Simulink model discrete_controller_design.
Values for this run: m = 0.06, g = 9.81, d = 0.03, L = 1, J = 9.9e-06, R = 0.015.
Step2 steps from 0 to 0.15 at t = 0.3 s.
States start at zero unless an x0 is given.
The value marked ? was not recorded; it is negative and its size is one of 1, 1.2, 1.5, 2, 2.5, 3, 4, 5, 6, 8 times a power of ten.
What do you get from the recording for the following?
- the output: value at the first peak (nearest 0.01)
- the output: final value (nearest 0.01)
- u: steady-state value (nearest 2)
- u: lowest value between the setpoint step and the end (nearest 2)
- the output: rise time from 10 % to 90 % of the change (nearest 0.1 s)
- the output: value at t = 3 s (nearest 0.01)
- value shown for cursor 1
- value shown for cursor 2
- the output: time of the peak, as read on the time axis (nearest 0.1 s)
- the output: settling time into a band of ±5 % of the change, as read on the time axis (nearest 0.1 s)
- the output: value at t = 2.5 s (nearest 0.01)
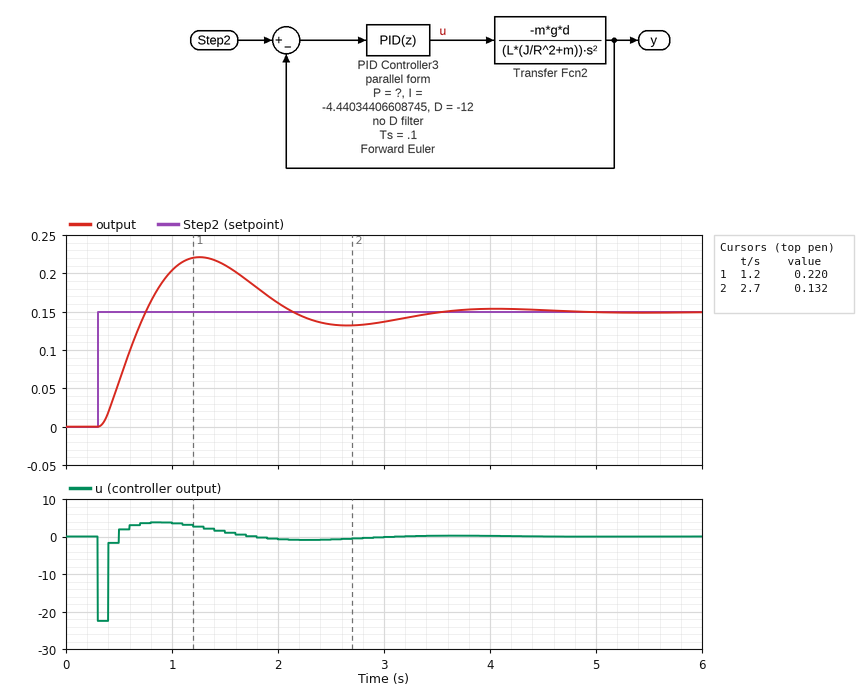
0.22
0.15
0
-22
0.3 s
0.14
0.220
0.132
1.3 s
3.2 s
0.13
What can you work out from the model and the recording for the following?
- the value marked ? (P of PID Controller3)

-30
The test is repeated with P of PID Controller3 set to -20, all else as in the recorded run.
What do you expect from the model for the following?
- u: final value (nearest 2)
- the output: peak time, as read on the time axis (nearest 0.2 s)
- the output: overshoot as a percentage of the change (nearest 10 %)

0
1.4 s
40 %
